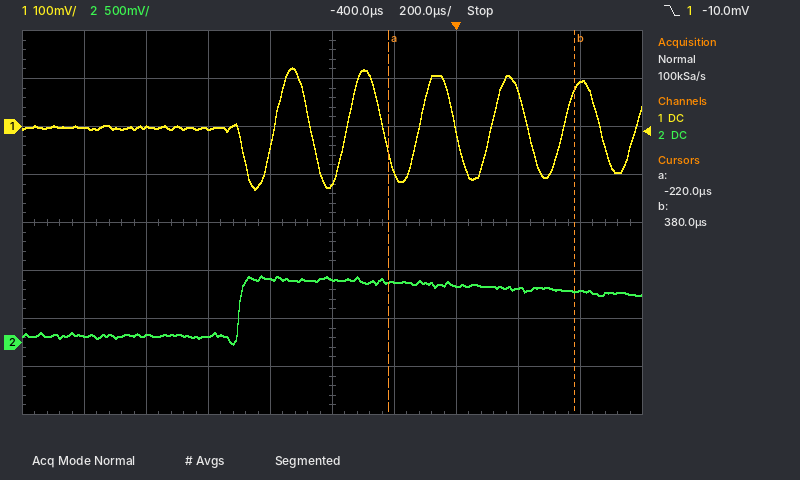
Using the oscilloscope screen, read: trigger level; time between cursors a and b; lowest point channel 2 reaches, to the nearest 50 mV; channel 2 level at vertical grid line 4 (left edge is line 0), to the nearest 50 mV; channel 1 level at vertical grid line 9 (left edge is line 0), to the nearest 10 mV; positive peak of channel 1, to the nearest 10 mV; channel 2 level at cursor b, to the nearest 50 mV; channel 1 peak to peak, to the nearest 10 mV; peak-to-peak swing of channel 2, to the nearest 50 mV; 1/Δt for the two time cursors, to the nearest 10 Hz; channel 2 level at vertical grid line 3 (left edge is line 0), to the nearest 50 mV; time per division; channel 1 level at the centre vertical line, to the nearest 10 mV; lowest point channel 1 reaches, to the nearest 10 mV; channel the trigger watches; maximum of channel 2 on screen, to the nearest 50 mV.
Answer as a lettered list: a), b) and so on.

a) -10.0 mV
b) 600 µs
c) 0 mV
d) 650 mV
e) 90 mV
f) 120 mV
g) 550 mV
h) 250 mV
i) 700 mV
j) 1.67 kHz
k) 50 mV
l) 200 µs
m) -120 mV
n) -130 mV
o) channel 1
p) 700 mV
